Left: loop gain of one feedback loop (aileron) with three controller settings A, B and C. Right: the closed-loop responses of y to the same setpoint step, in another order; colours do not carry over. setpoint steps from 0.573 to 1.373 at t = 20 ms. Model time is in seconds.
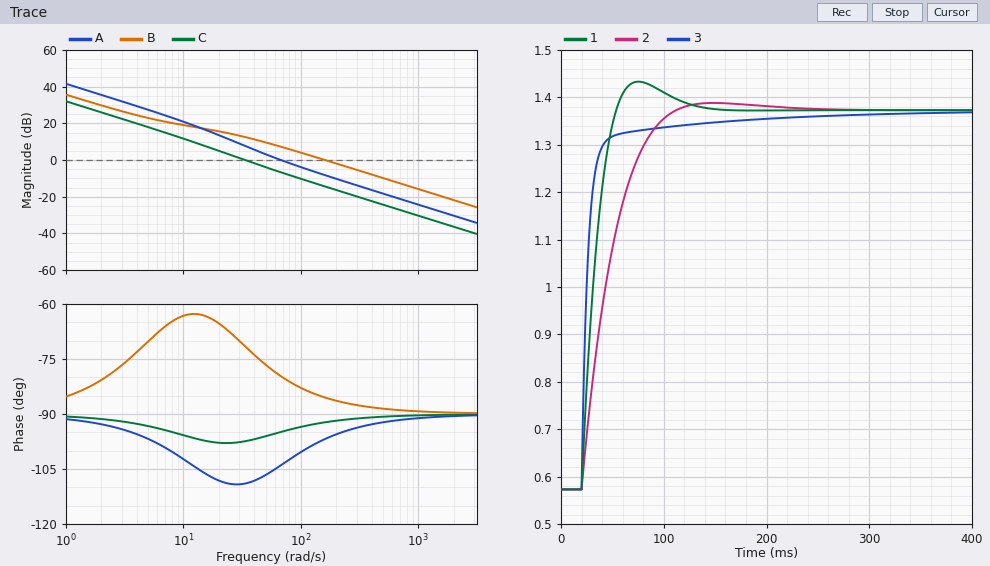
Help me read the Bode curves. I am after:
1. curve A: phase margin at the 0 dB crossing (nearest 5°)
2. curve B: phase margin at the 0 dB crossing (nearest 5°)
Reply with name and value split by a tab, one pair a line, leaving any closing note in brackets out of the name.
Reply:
curve A: phase margin at the 0 dB crossing	75°
curve B: phase margin at the 0 dB crossing	95°
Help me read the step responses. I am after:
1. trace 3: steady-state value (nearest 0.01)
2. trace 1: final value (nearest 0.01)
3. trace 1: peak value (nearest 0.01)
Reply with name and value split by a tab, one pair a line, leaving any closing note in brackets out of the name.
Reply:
trace 3: steady-state value	1.37
trace 1: final value	1.37
trace 1: peak value	1.43
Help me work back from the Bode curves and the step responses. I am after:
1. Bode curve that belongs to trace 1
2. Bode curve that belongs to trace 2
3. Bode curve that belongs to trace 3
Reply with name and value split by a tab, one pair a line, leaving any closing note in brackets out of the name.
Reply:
Bode curve that belongs to trace 1	A
Bode curve that belongs to trace 2	C
Bode curve that belongs to trace 3	B
